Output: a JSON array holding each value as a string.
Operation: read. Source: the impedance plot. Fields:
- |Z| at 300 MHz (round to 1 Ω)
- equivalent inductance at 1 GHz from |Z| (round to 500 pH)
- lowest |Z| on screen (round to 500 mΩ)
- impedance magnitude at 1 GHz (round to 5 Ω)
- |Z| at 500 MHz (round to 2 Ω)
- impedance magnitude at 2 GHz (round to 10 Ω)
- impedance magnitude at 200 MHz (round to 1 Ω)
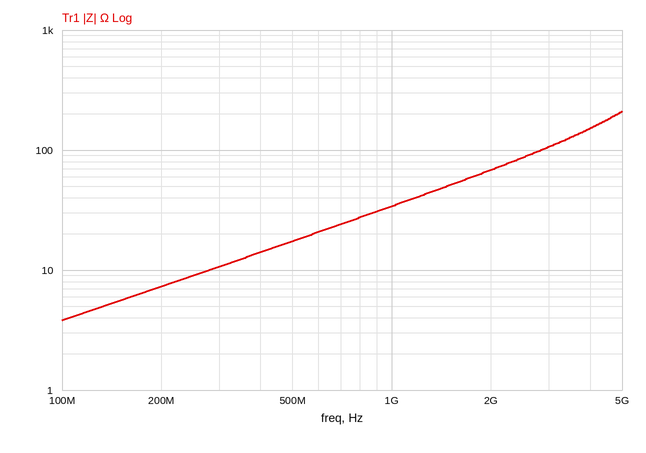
["11 Ω", "5.5 nH", "4.0 Ω", "35 Ω", "18 Ω", "70 Ω", "7 Ω"]
